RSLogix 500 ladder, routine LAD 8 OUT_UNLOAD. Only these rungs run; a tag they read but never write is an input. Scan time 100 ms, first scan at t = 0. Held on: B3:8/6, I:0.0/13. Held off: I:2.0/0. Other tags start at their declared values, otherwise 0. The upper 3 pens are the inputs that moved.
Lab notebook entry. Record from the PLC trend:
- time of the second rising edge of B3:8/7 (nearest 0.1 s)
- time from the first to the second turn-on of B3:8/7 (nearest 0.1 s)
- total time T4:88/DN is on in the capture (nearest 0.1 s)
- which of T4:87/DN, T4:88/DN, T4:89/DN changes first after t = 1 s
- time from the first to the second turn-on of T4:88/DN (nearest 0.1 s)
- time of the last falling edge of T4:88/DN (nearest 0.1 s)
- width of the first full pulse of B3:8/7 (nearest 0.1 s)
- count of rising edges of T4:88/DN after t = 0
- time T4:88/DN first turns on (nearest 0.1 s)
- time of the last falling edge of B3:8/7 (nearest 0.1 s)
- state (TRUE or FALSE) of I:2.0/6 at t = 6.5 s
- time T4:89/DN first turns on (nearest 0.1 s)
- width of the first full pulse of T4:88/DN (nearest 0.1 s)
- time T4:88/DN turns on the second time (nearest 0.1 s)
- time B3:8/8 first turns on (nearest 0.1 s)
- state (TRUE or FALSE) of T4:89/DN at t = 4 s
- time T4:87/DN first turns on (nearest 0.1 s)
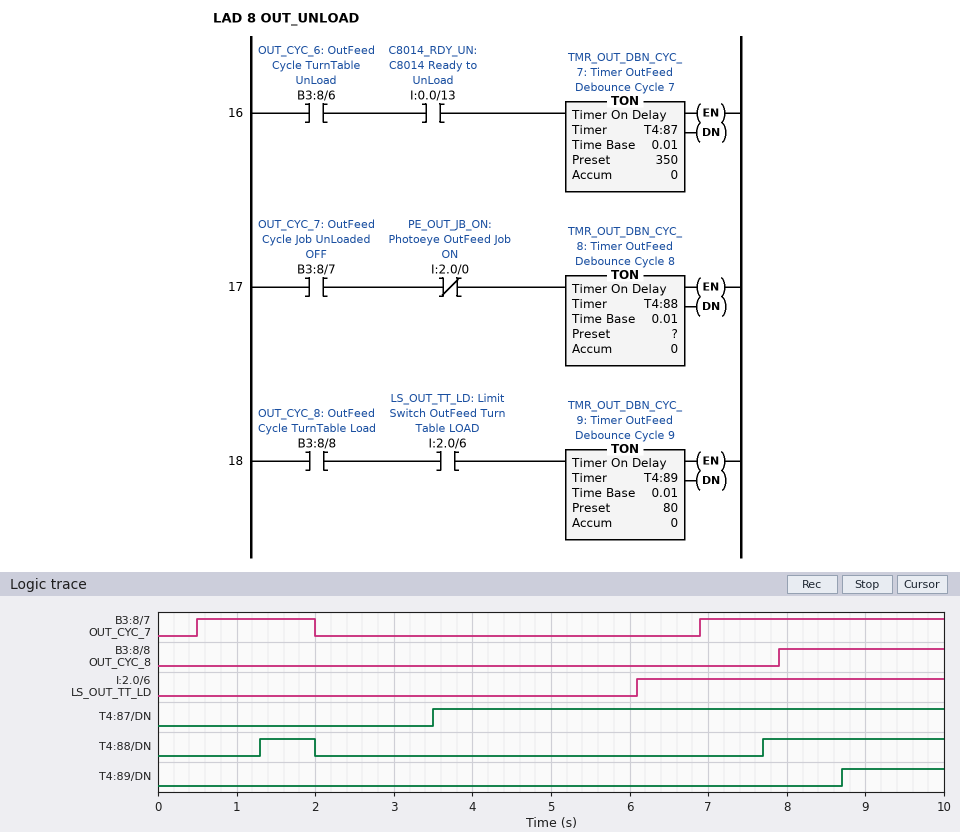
6.9 s
6.4 s
3.0 s
T4:88/DN
6.4 s
2.0 s
1.5 s
2
1.3 s
2.0 s
TRUE
8.7 s
0.7 s
7.7 s
7.9 s
FALSE
3.5 s
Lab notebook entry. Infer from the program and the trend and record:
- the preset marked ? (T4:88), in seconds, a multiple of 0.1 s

0.8 s
